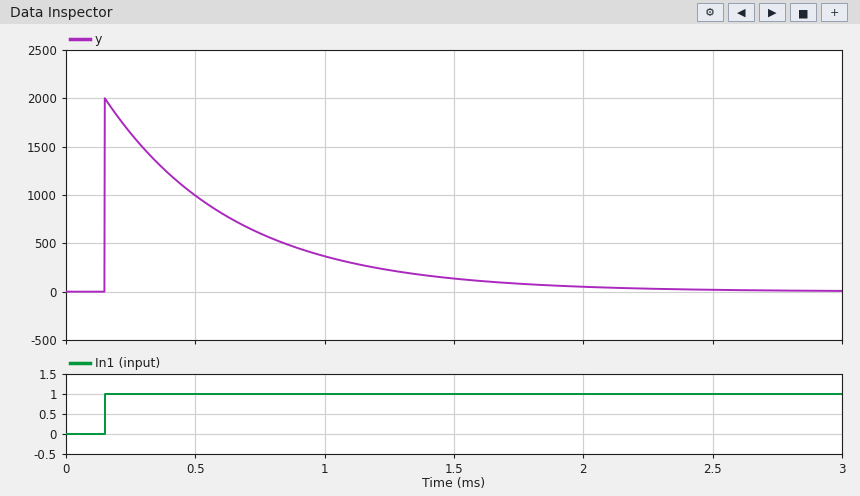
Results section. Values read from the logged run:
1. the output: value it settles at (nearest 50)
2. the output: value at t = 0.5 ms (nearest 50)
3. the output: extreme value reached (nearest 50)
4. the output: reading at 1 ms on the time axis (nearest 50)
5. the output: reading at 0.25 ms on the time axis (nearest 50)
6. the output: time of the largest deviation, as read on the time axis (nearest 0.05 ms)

0
1000
2000
350
1650
0.15 ms
